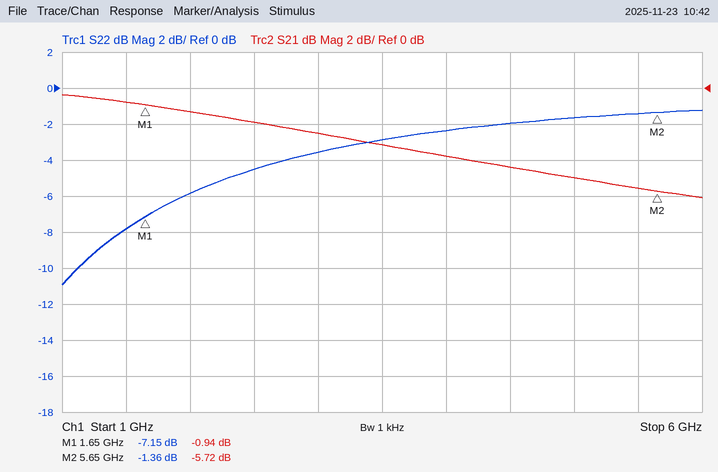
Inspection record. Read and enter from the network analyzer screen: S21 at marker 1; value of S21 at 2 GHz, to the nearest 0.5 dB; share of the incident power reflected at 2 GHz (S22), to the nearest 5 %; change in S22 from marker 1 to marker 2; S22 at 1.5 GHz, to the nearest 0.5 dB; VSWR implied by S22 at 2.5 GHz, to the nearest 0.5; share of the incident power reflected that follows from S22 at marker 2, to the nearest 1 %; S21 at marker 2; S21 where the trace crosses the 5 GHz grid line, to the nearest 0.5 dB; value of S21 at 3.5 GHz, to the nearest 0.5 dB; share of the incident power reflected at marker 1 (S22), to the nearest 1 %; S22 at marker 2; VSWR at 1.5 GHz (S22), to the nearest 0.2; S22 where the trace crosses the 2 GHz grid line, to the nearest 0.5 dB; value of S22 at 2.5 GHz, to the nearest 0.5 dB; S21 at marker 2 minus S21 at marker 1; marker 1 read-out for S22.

-0.94 dB
-1.5 dB
25 %
5.79 dB
-8.0 dB
4.0
73 %
-5.72 dB
-5.0 dB
-3.0 dB
19 %
-1.36 dB
2.4
-6.0 dB
-4.5 dB
-4.78 dB
-7.15 dB
